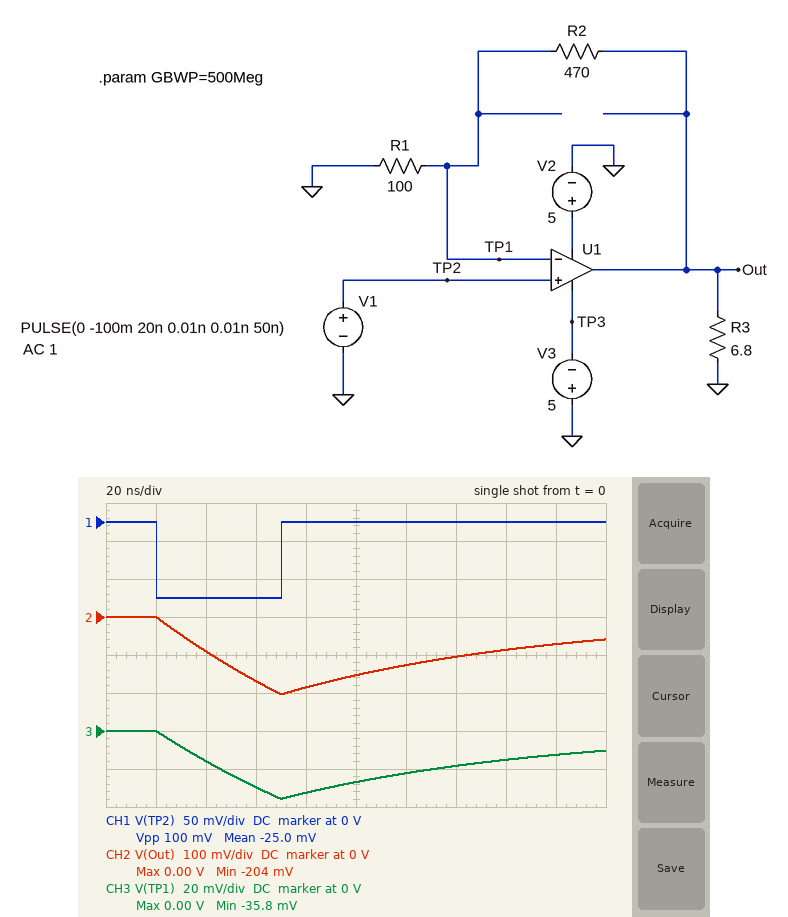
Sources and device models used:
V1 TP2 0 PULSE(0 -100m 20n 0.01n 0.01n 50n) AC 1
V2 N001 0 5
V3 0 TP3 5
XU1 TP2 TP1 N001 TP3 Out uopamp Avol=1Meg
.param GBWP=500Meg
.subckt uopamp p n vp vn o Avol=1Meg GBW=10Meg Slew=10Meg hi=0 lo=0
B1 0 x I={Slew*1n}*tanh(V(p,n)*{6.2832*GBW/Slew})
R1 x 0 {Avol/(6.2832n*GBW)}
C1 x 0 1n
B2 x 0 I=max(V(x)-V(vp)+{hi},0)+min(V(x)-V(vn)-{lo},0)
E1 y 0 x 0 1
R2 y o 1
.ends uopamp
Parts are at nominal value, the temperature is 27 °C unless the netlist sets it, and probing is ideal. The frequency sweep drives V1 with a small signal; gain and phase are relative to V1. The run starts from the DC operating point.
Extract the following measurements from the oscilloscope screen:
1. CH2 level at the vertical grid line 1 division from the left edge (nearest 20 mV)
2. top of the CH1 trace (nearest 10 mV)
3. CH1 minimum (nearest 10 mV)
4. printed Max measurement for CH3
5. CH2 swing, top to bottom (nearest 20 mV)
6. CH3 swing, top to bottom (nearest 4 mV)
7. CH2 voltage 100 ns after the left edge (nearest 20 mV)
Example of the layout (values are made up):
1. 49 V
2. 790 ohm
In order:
1. 0 V
2. 0 V
3. -100 mV
4. 0.00 V
5. 200 mV
6. 36 mV
7. -160 mV
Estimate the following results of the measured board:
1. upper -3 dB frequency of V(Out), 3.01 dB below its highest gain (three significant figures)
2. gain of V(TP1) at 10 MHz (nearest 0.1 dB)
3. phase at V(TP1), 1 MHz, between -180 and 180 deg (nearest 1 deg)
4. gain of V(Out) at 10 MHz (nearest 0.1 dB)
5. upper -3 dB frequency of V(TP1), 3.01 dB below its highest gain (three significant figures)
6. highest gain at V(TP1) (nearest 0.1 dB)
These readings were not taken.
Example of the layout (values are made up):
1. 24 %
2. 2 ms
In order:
1. 1.53 MHz
2. -16.4 dB
3. -33 deg
4. -1.3 dB
5. 1.53 MHz
6. 0 dB
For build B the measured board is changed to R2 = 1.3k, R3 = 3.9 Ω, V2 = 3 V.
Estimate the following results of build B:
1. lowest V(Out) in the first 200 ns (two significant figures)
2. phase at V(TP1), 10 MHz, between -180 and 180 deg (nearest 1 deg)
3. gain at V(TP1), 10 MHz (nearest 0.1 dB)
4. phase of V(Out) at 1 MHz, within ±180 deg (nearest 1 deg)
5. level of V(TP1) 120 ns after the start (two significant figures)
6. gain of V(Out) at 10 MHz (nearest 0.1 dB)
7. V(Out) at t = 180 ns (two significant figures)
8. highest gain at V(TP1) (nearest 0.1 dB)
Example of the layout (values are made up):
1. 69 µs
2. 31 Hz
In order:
1. -210 mV
2. -87 deg
3. -24.9 dB
4. -60 deg
5. -12 mV
6. -2.0 dB
7. -140 mV
8. 0 dB
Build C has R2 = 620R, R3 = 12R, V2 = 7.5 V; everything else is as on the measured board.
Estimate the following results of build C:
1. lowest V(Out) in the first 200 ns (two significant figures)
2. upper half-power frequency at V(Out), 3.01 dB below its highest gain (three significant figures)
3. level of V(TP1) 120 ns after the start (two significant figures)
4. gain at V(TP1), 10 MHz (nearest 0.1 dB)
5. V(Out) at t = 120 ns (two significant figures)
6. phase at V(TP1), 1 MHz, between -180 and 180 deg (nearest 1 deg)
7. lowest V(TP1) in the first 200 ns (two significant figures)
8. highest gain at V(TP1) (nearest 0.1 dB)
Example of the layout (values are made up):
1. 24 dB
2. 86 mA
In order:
1. -220 mV
2. 1.28 MHz
3. -21 mV
4. -17.9 dB
5. -150 mV
6. -38 deg
7. -31 mV
8. 0 dB
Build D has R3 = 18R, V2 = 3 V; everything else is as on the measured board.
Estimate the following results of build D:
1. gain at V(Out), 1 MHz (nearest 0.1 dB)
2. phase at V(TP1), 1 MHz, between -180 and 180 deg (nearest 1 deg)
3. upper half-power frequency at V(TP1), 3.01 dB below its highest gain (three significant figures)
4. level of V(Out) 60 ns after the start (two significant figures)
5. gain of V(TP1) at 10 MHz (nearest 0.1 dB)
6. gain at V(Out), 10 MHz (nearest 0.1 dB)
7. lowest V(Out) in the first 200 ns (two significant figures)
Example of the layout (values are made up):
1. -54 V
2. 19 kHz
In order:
1. 13.8 dB
2. -31 deg
3. 1.66 MHz
4. -180 mV
5. -15.7 dB
6. -0.6 dB
7. -220 mV
